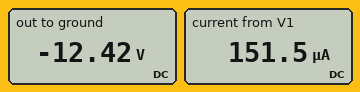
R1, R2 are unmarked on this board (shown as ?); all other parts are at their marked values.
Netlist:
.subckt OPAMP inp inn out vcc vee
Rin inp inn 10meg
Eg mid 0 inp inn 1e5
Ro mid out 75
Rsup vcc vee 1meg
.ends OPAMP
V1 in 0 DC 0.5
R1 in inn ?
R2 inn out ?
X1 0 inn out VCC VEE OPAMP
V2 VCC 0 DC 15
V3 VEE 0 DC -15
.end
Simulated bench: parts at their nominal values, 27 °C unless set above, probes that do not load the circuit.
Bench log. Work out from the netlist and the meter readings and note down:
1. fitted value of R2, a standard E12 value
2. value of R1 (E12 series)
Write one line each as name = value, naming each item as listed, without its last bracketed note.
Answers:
fitted value of R2, a standard E12 value = 82 kΩ
value of R1 = 3.3 kΩ
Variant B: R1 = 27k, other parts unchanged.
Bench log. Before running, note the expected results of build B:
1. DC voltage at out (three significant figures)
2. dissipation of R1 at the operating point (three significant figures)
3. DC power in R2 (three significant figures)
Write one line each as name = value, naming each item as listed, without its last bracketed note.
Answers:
DC voltage at out = -1.52 V
dissipation of R1 at the operating point = 9.26 µW
DC power in R2 = 28.1 µW
